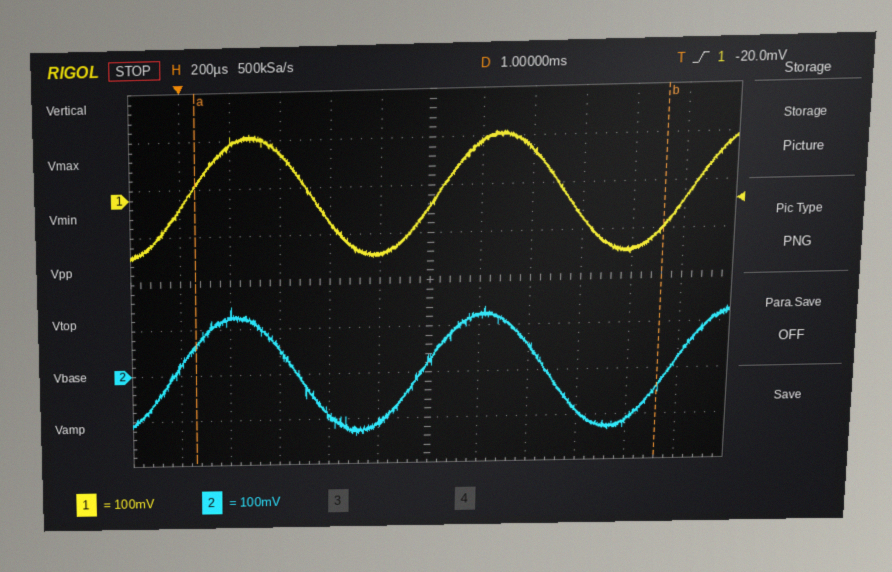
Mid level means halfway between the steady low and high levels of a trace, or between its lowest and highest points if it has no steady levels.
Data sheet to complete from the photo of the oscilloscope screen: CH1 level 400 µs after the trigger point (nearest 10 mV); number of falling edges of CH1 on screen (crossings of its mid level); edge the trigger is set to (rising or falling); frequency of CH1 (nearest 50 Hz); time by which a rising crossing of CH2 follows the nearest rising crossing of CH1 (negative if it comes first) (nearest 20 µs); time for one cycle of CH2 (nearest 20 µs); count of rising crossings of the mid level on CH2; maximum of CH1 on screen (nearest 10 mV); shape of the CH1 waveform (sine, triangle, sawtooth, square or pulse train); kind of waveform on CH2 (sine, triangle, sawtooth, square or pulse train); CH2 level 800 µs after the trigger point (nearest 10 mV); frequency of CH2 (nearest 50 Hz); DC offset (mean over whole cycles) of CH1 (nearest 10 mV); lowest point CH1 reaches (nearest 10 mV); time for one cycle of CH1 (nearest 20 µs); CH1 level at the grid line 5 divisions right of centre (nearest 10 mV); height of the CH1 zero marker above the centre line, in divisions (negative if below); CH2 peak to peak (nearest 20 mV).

90 mV
2
rising
1.00 kHz
-40 µs
1.00 ms
3
130 mV
sine
sine
-110 mV
1.00 kHz
0 mV
-130 mV
1.00 ms
-20 mV
+1.8 div
280 mV
